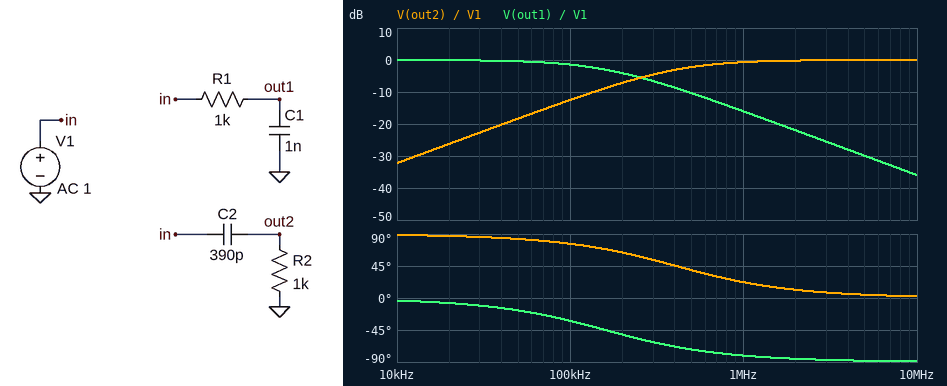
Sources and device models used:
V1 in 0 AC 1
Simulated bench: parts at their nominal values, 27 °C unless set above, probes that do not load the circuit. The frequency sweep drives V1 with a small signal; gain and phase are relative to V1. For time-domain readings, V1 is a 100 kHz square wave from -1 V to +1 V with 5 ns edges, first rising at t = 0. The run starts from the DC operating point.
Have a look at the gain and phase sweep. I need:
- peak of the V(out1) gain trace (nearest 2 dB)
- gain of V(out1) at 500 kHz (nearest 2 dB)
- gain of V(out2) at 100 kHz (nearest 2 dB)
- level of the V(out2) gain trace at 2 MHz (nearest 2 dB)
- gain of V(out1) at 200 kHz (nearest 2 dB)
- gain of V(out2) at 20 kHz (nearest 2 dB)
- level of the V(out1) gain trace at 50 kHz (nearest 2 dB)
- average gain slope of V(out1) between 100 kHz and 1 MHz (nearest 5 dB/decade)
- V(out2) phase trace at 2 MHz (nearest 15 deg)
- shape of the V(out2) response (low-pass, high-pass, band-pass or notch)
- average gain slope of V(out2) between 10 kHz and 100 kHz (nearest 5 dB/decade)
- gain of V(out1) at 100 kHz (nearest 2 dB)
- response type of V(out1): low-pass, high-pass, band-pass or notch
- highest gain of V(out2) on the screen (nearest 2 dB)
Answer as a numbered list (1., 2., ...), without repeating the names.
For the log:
1. 0 dB
2. -10 dB
3. -12 dB
4. 0 dB
5. -4 dB
6. -26 dB
7. 0 dB
8. -15 dB/decade
9. 15 deg
10. high-pass
11. 20 dB/decade
12. -2 dB
13. low-pass
14. 0 dB
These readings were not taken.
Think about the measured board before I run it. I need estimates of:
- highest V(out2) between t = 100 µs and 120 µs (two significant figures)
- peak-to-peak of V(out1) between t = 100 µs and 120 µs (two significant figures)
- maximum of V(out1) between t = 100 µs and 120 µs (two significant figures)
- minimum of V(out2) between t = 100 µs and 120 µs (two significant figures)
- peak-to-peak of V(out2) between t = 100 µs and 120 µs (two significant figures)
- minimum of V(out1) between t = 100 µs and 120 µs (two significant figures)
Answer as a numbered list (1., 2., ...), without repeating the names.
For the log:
1. 2.0 V
2. 2.0 V
3. 990 mV
4. -2.0 V
5. 4.0 V
6. -990 mV
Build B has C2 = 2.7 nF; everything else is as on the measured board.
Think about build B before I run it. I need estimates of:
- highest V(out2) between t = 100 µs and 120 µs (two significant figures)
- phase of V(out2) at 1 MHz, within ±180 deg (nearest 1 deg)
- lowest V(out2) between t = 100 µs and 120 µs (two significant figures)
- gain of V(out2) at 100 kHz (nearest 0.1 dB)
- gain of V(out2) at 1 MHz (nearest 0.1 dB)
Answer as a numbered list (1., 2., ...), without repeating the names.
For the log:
1. 1.7 V
2. 3 deg
3. -1.7 V
4. -1.3 dB
5. 0 dB
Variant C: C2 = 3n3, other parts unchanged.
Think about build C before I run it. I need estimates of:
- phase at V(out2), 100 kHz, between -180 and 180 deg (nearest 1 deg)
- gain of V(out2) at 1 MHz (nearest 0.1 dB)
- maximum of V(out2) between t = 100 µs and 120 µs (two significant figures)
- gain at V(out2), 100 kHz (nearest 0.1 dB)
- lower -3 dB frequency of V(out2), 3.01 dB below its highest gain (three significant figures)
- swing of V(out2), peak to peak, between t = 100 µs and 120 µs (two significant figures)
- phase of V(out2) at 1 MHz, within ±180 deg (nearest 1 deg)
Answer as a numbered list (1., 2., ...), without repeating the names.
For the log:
1. 26 deg
2. 0 dB
3. 1.6 V
4. -0.9 dB
5. 48.2 kHz
6. 3.3 V
7. 3 deg
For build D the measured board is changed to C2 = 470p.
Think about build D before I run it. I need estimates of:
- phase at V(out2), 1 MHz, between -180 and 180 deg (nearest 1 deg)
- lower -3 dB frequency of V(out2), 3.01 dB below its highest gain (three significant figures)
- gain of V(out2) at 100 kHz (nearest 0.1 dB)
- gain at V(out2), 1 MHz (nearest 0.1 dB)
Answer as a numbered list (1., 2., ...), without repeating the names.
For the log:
1. 19 deg
2. 339 kHz
3. -11.0 dB
4. -0.5 dB
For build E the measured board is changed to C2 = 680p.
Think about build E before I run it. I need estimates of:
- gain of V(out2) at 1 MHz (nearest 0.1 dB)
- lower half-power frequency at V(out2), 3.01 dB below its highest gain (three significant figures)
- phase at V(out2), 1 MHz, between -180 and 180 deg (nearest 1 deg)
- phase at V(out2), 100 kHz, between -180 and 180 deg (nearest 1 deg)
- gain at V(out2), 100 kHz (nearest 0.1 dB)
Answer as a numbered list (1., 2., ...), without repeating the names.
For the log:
1. -0.2 dB
2. 234 kHz
3. 13 deg
4. 67 deg
5. -8.1 dB
